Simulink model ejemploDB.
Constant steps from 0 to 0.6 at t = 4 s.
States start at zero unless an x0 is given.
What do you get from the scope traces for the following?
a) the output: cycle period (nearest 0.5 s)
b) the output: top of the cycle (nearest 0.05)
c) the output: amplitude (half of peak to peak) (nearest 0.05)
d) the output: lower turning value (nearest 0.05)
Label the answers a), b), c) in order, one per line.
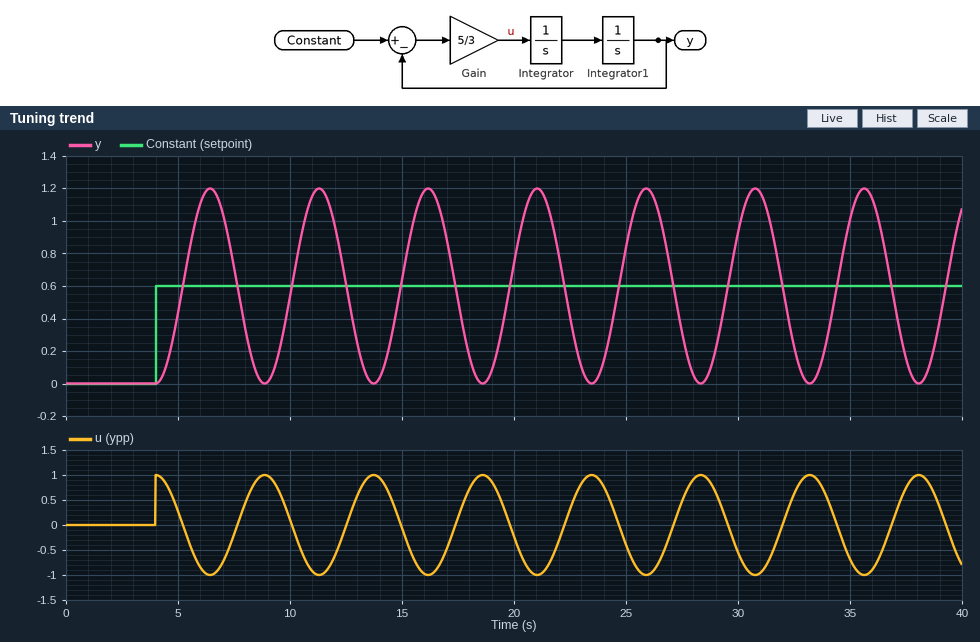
a) 5.0 s
b) 1.20
c) 0.60
d) 0.00
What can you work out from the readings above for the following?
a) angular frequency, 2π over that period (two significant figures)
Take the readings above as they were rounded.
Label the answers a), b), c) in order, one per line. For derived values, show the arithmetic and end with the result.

a) 2π / 5 = 1.3 rad/s
